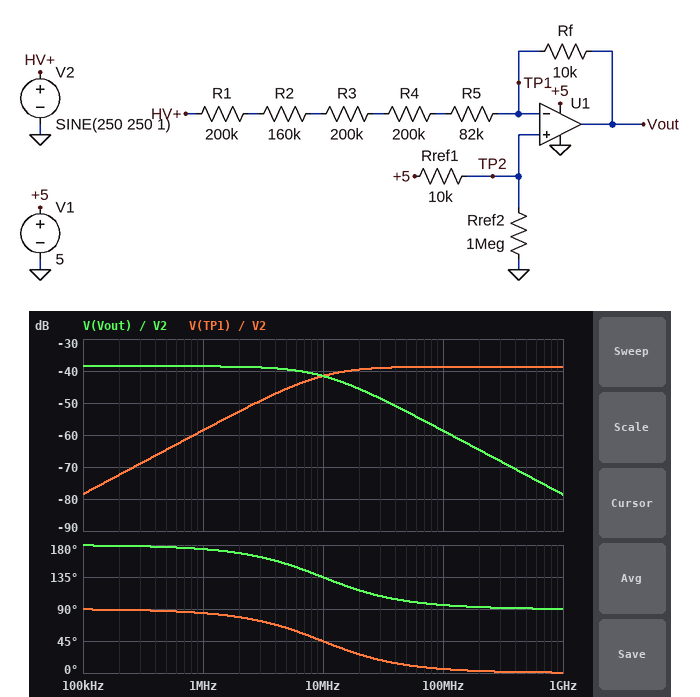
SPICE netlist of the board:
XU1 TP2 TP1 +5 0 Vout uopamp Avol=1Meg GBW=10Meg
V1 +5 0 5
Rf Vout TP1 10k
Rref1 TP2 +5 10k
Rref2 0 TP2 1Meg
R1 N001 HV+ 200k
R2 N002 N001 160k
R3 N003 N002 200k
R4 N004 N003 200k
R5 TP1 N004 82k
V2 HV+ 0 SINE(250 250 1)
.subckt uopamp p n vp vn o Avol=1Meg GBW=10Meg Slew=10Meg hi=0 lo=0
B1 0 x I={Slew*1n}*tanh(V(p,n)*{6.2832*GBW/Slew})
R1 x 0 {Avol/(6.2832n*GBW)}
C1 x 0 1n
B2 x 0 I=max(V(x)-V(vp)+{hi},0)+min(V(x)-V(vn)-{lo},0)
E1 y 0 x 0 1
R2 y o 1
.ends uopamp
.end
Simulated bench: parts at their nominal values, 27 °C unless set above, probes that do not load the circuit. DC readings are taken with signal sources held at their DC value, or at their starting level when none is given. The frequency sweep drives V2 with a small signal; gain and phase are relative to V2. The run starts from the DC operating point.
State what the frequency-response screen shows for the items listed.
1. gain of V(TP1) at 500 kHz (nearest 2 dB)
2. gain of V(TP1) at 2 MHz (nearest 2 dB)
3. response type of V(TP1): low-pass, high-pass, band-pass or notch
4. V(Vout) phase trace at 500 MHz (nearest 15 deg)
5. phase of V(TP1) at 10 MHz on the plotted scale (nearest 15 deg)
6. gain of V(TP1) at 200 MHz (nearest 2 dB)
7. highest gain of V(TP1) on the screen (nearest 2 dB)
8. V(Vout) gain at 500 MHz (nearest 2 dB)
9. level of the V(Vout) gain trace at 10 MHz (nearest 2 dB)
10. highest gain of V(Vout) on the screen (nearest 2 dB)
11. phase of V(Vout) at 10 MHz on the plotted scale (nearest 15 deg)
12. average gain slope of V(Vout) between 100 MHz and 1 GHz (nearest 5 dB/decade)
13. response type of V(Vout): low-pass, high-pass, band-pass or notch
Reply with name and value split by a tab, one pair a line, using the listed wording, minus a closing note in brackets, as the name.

gain of V(TP1) at 500 kHz	-64 dB
gain of V(TP1) at 2 MHz	-52 dB
response type of V(TP1): low-pass, high-pass, band-pass or notch	high-pass
V(Vout) phase trace at 500 MHz	90 deg
phase of V(TP1) at 10 MHz on the plotted scale	45 deg
gain of V(TP1) at 200 MHz	-38 dB
highest gain of V(TP1) on the screen	-38 dB
V(Vout) gain at 500 MHz	-72 dB
level of the V(Vout) gain trace at 10 MHz	-42 dB
highest gain of V(Vout) on the screen	-38 dB
phase of V(Vout) at 10 MHz on the plotted scale	135 deg
average gain slope of V(Vout) between 100 MHz and 1 GHz	-20 dB/decade
response type of V(Vout): low-pass, high-pass, band-pass or notch	low-pass
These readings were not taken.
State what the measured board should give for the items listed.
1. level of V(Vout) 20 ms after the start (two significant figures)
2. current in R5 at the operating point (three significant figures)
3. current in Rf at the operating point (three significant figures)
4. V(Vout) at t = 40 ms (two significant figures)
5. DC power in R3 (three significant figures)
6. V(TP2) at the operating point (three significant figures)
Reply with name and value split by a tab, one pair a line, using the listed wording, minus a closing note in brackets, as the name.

level of V(Vout) 20 ms after the start	1.7 V
current in R5 at the operating point	291 µA
current in Rf at the operating point	291 µA
V(Vout) at t = 40 ms	1.3 V
DC power in R3	16.9 mW
V(TP2) at the operating point	4.95 V
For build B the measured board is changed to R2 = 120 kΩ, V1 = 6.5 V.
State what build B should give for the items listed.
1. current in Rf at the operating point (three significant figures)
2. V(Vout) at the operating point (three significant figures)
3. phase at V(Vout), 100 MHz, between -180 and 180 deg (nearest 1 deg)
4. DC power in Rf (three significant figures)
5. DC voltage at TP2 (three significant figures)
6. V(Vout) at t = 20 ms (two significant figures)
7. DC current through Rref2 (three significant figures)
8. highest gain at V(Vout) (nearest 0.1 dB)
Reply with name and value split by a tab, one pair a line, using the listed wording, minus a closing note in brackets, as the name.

current in Rf at the operating point	304 µA
V(Vout) at the operating point	3.40 V
phase at V(Vout), 100 MHz, between -180 and 180 deg	96 deg
DC power in Rf	922 µW
DC voltage at TP2	6.44 V
V(Vout) at t = 20 ms	3.0 V
DC current through Rref2	6.44 µA
highest gain at V(Vout)	-38.1 dB
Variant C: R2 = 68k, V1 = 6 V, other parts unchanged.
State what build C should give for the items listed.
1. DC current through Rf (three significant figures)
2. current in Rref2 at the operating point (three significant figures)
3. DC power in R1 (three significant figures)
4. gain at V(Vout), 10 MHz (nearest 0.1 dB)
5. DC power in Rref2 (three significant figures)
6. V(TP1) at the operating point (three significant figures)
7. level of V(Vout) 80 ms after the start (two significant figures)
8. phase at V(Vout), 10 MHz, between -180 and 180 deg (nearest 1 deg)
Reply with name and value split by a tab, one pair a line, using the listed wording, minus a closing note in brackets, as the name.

DC current through Rf	325 µA
current in Rref2 at the operating point	5.94 µA
DC power in R1	21.2 mW
gain at V(Vout), 10 MHz	-40.6 dB
DC power in Rref2	35.3 µW
V(TP1) at the operating point	5.94 V
level of V(Vout) 80 ms after the start	1.1 V
phase at V(Vout), 10 MHz, between -180 and 180 deg	135 deg
